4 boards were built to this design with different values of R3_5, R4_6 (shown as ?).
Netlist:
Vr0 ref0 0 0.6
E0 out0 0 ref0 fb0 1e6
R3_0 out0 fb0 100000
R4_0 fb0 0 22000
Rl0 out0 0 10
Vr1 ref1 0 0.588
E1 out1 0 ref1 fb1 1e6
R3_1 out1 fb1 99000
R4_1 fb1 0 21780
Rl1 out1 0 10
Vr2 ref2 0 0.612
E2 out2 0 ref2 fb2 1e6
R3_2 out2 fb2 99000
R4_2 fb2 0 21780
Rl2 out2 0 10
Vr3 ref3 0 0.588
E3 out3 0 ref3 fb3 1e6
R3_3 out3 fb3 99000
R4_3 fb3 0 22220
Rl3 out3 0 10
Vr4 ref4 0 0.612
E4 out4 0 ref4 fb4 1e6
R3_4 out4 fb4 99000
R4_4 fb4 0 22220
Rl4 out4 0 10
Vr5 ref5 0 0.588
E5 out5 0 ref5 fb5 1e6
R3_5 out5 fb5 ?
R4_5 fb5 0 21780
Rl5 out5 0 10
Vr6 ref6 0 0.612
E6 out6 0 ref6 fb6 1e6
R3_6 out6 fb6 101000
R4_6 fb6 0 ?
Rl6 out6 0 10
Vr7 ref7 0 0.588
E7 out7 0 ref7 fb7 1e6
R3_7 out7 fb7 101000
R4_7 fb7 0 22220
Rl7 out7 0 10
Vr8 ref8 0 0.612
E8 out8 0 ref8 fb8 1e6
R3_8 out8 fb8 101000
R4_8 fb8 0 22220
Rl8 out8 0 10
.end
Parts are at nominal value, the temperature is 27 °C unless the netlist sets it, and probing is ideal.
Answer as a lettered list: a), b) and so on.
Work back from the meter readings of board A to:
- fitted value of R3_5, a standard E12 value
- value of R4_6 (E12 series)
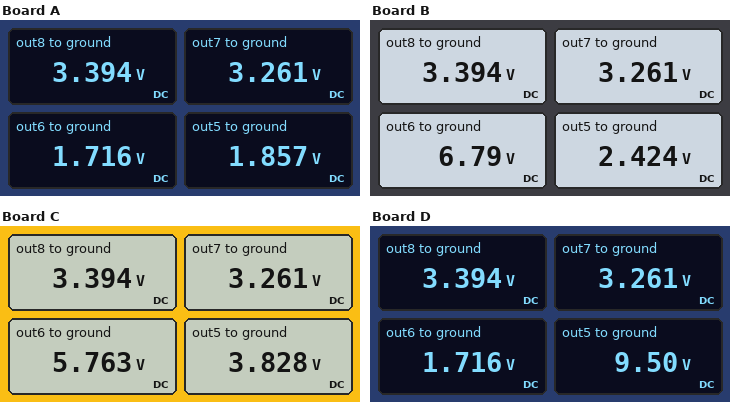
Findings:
a) 47 kΩ
b) 56 kΩ
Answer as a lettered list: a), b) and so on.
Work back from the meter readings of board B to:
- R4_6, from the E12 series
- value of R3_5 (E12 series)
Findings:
a) 10 kΩ
b) 68 kΩ
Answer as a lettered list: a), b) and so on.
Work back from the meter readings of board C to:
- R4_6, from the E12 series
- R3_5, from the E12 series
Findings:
a) 12 kΩ
b) 120 kΩ
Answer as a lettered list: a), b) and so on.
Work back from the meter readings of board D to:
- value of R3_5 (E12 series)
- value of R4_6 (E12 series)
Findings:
a) 330 kΩ
b) 56 kΩ
